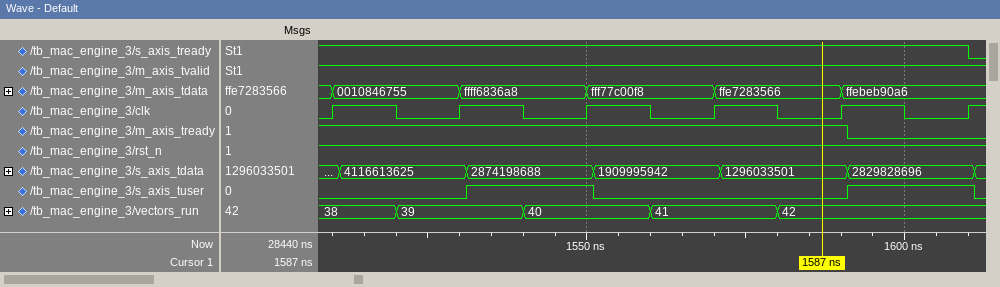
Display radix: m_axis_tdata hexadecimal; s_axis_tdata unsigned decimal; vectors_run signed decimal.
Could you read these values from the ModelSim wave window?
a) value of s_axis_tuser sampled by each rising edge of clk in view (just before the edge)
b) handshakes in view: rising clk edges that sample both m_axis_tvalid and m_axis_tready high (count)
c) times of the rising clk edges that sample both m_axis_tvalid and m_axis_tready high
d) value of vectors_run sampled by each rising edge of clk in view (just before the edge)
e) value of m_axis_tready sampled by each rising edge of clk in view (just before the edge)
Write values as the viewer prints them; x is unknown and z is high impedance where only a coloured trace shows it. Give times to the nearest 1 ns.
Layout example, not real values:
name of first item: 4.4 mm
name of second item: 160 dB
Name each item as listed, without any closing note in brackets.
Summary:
value of s_axis_tuser sampled by each rising edge of clk in view: 0 0 1 0 0 1
handshakes in view: rising clk edges that sample both m_axis_tvalid and m_axis_tready high: 5
times of the rising clk edges that sample both m_axis_tvalid and m_axis_tready high: 1510 ns, 1530 ns, 1550 ns, 1570 ns, 1590 ns
value of vectors_run sampled by each rising edge of clk in view: 38, 39, 40, 41, 42, 42
value of m_axis_tready sampled by each rising edge of clk in view: 1 1 1 1 1 0
